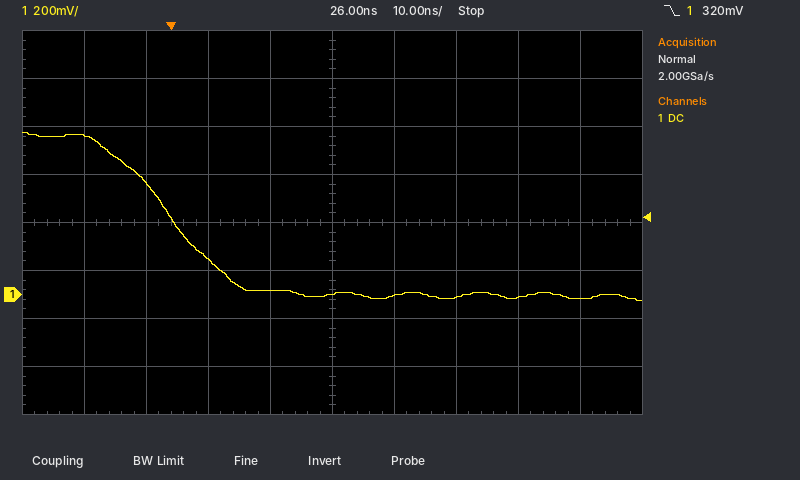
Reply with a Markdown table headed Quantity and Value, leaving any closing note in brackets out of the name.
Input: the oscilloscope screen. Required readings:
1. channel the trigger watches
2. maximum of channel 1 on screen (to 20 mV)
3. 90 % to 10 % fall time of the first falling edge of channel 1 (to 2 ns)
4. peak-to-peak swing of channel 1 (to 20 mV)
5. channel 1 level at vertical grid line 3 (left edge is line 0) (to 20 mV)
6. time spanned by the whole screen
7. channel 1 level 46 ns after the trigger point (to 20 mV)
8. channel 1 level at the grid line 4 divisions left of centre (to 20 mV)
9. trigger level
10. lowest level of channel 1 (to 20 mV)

| Quantity | Value |
|---|---|
| channel the trigger watches | channel 1 |
| maximum of channel 1 on screen | 680 mV |
| 90 % to 10 % fall time of the first falling edge of channel 1 | 20 ns |
| peak-to-peak swing of channel 1 | 700 mV |
| channel 1 level at vertical grid line 3 (left edge is line 0) | 140 mV |
| time spanned by the whole screen | 100 ns |
| channel 1 level 46 ns after the trigger point | -20 mV |
| channel 1 level at the grid line 4 divisions left of centre | 660 mV |
| trigger level | 320 mV |
| lowest level of channel 1 | -20 mV |
